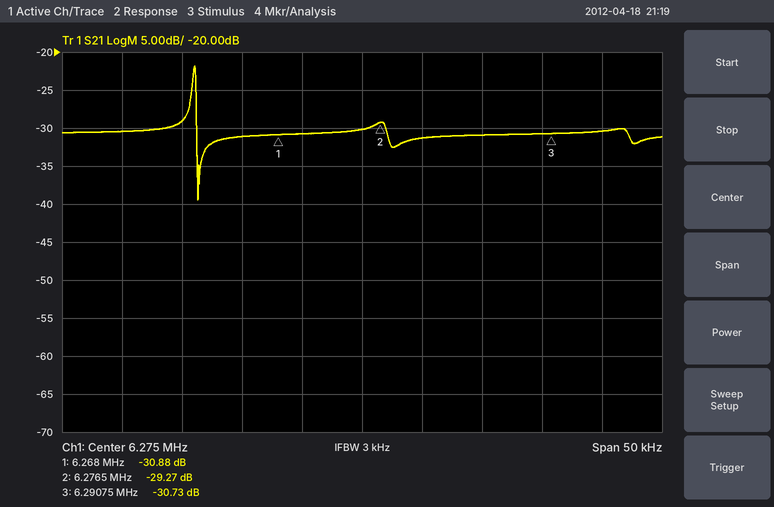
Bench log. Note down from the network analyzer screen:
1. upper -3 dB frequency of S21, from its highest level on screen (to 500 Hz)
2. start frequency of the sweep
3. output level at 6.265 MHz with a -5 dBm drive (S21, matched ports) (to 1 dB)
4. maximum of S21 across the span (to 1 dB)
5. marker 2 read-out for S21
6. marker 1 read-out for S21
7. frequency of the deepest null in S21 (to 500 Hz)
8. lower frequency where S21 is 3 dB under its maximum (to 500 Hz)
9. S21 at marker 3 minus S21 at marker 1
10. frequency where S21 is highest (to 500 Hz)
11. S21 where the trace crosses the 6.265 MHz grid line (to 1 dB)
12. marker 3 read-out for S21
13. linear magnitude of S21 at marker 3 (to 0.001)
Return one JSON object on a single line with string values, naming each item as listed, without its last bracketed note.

{"upper -3 dB frequency of S21, from its highest level on screen": "6.2610 MHz", "start frequency of the sweep": "6.25 MHz", "output level at 6.265 MHz with a -5 dBm drive (S21, matched ports)": "-36 dBm", "maximum of S21 across the span": "-22 dB", "marker 2 read-out for S21": "-29.27 dB", "marker 1 read-out for S21": "-30.88 dB", "frequency of the deepest null in S21": "6.2615 MHz", "lower frequency where S21 is 3 dB under its maximum": "6.2610 MHz", "S21 at marker 3 minus S21 at marker 1": "0.15 dB", "frequency where S21 is highest": "6.2610 MHz", "S21 where the trace crosses the 6.265 MHz grid line": "-31 dB", "marker 3 read-out for S21": "-30.73 dB", "linear magnitude of S21 at marker 3": "0.029"}
